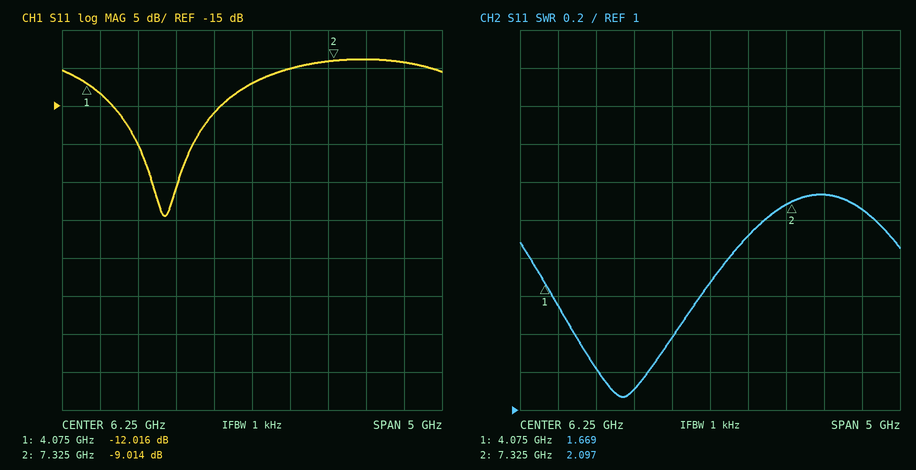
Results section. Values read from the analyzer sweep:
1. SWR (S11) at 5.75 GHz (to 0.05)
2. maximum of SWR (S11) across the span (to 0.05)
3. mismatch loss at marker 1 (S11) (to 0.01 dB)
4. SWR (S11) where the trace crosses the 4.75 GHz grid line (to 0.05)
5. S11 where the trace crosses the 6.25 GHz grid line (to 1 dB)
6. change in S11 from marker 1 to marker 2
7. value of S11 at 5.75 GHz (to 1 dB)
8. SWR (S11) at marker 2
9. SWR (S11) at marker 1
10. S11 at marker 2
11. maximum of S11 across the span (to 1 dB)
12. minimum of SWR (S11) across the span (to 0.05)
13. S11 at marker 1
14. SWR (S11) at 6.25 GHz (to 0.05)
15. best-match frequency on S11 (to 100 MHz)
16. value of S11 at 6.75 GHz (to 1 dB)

1.40
2.15
0.28 dB
1.20
-12 dB
3.002 dB
-16 dB
2.097
1.669
-9.014 dB
-9 dB
1.05
-12.016 dB
1.65
5.1 GHz
-10 dB
